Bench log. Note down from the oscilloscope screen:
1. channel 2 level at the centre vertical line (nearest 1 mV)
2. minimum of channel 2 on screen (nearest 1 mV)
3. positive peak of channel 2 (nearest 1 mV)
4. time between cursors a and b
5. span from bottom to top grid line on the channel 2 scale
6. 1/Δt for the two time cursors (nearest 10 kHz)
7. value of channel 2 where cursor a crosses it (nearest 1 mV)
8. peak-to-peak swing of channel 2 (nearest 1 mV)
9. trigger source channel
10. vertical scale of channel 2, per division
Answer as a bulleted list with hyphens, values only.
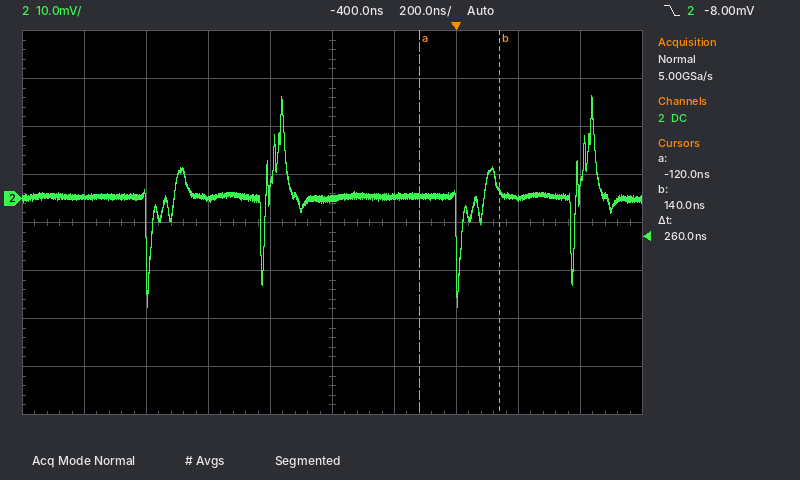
- 0 mV
- -23 mV
- 21 mV
- 260 ns
- 80 mV
- 3.85 MHz
- 0 mV
- 44 mV
- channel 2
- 10 mV
